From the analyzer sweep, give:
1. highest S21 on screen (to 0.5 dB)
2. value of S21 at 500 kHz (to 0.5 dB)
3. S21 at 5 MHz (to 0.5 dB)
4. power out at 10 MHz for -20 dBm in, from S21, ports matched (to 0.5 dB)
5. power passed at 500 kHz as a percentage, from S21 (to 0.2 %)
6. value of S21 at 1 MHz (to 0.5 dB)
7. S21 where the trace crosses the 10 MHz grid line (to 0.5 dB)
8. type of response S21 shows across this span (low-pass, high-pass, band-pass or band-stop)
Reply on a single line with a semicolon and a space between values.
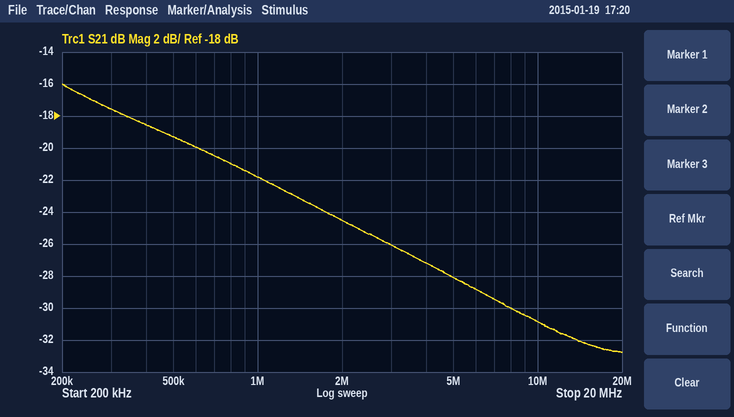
-16.0 dB; -19.5 dB; -28.0 dB; -51.0 dBm; 1.2 %; -22.0 dB; -31.0 dB; low-pass
